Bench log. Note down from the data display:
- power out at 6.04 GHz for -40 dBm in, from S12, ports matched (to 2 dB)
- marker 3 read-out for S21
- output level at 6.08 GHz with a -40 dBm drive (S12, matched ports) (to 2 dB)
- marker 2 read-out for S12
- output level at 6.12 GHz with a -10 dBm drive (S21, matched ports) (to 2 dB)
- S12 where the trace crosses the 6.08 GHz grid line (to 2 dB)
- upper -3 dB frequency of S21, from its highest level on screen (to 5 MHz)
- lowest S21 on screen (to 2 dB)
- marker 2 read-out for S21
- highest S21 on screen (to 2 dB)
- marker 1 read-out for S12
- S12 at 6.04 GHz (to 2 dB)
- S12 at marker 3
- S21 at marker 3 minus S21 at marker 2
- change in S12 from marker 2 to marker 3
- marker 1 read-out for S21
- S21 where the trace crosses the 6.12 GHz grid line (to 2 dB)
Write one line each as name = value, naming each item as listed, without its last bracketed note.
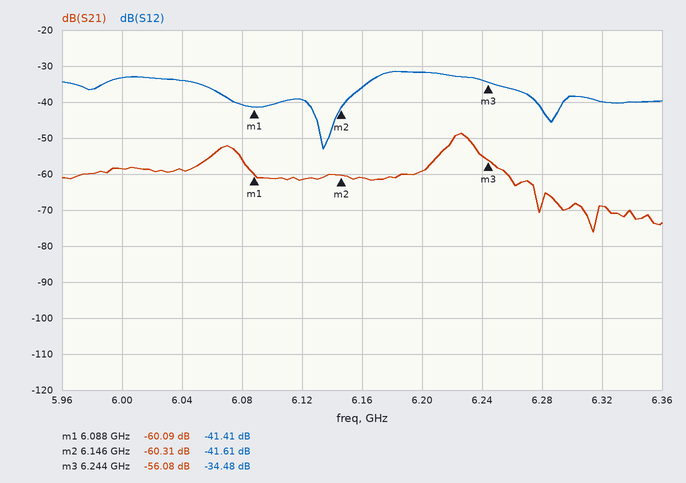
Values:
power out at 6.04 GHz for -40 dBm in, from S12, ports matched = -74 dBm
marker 3 read-out for S21 = -56.08 dB
output level at 6.08 GHz with a -40 dBm drive (S12, matched ports) = -80 dBm
marker 2 read-out for S12 = -41.61 dB
output level at 6.12 GHz with a -10 dBm drive (S21, matched ports) = -72 dBm
S12 where the trace crosses the 6.08 GHz grid line = -40 dB
upper -3 dB frequency of S21, from its highest level on screen = 6.235 GHz
lowest S21 on screen = -76 dB
marker 2 read-out for S21 = -60.31 dB
highest S21 on screen = -48 dB
marker 1 read-out for S12 = -41.41 dB
S12 at 6.04 GHz = -34 dB
S12 at marker 3 = -34.48 dB
S21 at marker 3 minus S21 at marker 2 = 4.23 dB
change in S12 from marker 2 to marker 3 = 7.13 dB
marker 1 read-out for S21 = -60.09 dB
S21 where the trace crosses the 6.12 GHz grid line = -62 dB
